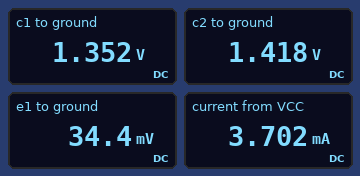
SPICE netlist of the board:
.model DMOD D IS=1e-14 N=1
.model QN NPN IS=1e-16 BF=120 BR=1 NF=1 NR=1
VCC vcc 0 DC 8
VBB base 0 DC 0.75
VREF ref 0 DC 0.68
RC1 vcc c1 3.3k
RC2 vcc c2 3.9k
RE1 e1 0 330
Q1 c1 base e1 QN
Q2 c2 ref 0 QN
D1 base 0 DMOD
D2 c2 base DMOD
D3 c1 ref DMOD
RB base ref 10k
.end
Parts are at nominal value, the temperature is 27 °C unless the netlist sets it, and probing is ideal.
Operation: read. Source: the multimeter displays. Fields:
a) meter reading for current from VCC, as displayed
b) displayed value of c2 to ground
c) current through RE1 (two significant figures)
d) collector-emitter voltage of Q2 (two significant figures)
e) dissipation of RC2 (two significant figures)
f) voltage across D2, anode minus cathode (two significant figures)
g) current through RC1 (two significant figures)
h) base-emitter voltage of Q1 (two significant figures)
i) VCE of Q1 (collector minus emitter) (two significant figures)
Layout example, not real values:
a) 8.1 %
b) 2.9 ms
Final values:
a) 3.702 mA
b) 1.418 V
c) 100 µA
d) 1.4 V
e) 11 mW
f) 670 mV
g) 2.0 mA
h) 720 mV
i) 1.3 V
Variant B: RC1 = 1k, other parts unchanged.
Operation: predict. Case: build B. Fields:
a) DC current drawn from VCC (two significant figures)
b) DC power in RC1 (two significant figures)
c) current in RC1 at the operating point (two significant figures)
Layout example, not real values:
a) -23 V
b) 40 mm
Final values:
a) 8.3 mA
b) 44 mW
c) 6.6 mA
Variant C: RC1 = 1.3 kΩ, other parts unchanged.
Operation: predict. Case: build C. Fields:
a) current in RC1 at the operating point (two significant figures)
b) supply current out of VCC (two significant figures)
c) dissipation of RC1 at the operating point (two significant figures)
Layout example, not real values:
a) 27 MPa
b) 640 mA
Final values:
a) 5.1 mA
b) 6.8 mA
c) 34 mW
